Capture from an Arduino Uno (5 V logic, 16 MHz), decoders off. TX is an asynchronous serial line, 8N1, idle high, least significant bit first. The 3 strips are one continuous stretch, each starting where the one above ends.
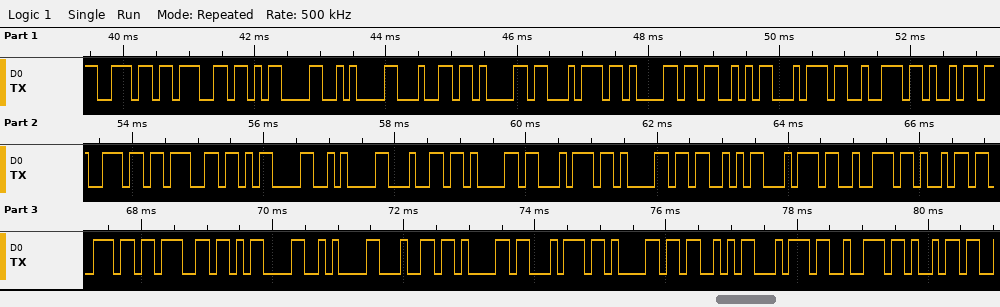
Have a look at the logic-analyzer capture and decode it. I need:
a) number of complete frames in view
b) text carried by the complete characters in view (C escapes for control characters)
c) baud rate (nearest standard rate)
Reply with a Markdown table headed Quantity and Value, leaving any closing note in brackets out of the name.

| Quantity | Value |
|---|---|
| number of complete frames in view | 36 |
| text carried by the complete characters in view | "ng\r\ndataString\r\ndataString\r\ndataStri" |
| baud rate | 9600 baud |
